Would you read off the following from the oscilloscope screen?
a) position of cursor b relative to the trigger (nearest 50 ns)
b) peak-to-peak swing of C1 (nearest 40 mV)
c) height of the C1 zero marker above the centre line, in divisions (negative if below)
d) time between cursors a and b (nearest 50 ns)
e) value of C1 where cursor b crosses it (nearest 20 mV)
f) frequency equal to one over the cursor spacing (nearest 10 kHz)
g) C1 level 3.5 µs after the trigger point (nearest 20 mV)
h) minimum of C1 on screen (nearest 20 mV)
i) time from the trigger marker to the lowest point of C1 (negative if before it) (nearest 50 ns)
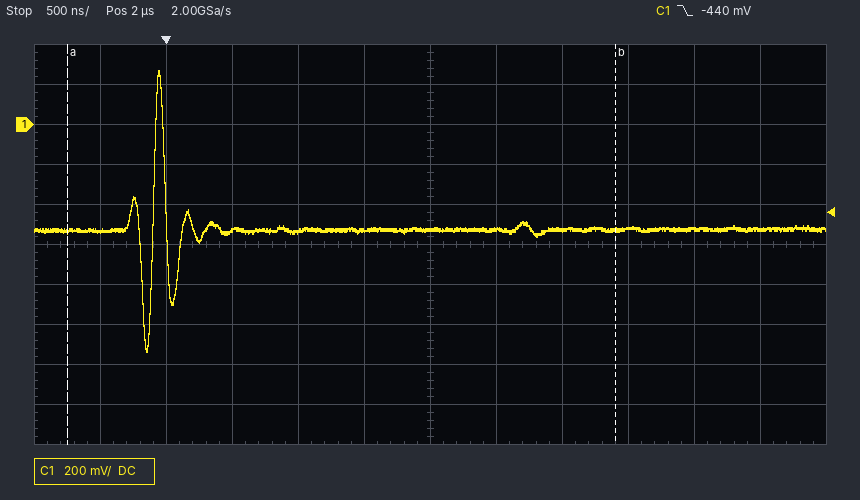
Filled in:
+3.40 µs
1.40 V
+3.0 div
4.15 µs
-520 mV
240 kHz
-520 mV
-1.14 V
-150 ns
